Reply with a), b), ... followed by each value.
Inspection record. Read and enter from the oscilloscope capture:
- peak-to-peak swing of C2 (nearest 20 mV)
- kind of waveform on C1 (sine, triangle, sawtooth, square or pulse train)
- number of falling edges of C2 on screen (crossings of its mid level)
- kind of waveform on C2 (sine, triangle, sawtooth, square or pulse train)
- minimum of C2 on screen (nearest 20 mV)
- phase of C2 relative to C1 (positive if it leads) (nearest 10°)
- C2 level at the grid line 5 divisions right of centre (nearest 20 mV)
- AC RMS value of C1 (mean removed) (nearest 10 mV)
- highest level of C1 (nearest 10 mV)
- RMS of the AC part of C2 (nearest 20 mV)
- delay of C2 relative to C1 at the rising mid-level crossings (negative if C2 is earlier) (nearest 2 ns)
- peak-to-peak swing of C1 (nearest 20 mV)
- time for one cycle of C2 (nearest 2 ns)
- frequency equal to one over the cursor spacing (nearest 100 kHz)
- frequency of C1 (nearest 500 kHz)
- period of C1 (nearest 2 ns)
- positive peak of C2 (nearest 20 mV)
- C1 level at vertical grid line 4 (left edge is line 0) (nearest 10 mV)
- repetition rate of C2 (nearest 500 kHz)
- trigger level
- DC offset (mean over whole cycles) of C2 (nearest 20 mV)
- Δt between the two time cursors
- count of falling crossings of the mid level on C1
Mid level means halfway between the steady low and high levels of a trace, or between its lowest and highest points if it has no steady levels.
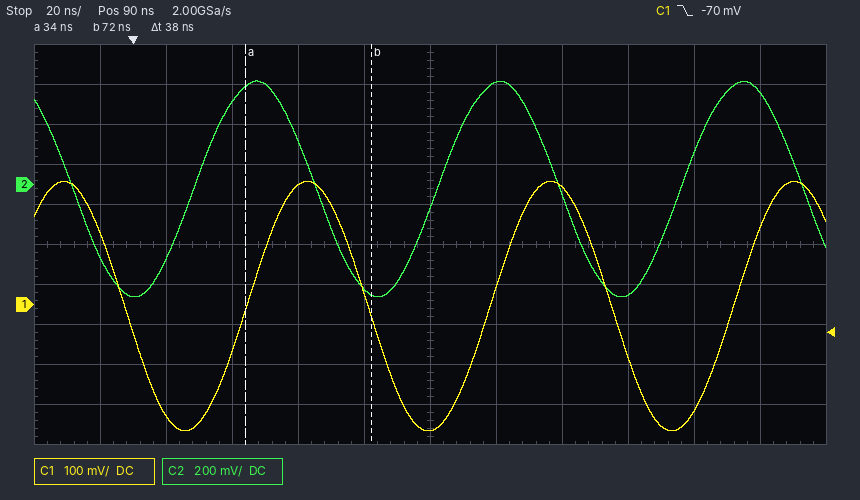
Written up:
a) 1.08 V
b) sine
c) 4
d) sine
e) -560 mV
f) +80°
g) 460 mV
h) 220 mV
i) 310 mV
j) 380 mV
k) -16 ns
l) 620 mV
m) 74 ns
n) 26.3 MHz
o) 13.5 MHz
p) 74 ns
q) 520 mV
r) 300 mV
s) 13.5 MHz
t) -70 mV
u) -20 mV
v) 38 ns
w) 3
